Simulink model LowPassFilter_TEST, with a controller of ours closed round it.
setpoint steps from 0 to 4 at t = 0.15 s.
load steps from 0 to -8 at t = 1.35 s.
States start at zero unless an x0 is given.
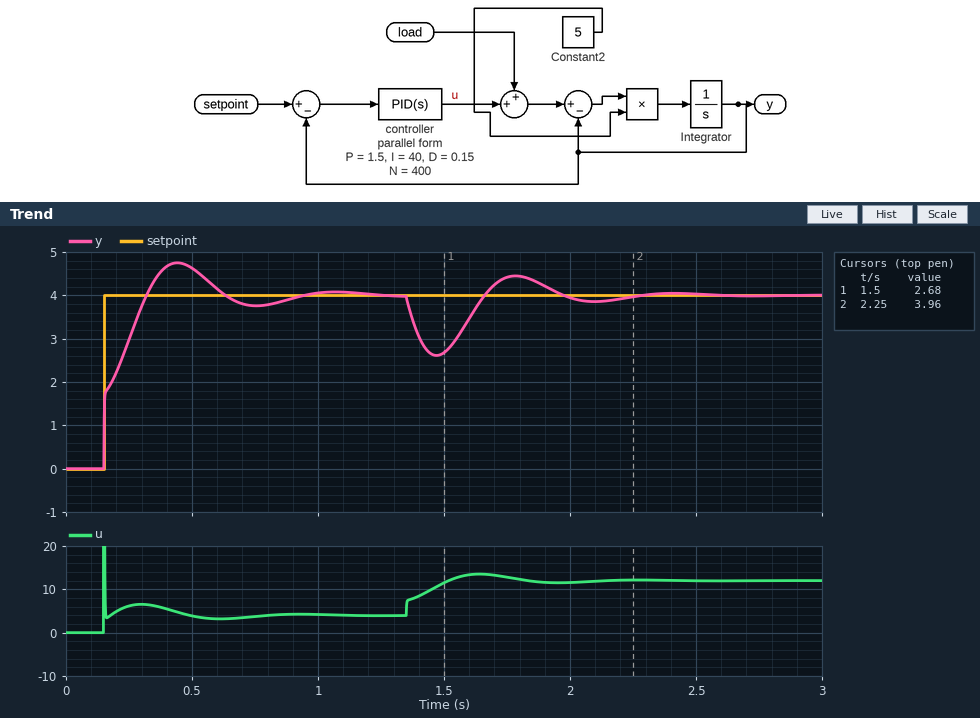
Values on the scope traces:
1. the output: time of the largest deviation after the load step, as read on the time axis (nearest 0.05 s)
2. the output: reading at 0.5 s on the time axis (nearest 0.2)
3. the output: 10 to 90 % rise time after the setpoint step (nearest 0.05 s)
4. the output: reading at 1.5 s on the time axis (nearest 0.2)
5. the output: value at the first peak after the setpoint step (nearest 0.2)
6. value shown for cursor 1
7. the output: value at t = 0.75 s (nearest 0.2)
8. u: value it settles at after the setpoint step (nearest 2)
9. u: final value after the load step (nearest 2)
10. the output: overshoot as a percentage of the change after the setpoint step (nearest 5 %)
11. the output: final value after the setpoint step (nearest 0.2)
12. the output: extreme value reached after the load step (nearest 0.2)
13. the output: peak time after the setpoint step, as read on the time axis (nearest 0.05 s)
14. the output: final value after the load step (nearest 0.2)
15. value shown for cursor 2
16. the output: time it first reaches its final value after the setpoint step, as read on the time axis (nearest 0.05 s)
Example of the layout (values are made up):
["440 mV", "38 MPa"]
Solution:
["1.45 s", "4.6", "0.15 s", "2.6", "4.8", "2.68", "3.8", "4", "12", "20 %", "4.0", "2.6", "0.45 s", "4.0", "3.96", "0.30 s"]
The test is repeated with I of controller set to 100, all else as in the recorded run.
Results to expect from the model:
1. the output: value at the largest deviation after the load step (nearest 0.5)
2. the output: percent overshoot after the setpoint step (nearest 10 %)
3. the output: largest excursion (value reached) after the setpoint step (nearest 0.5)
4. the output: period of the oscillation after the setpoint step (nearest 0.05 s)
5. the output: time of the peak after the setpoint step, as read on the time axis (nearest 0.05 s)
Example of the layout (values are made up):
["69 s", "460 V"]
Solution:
["3.0", "30 %", "5.0", "0.40 s", "0.35 s"]
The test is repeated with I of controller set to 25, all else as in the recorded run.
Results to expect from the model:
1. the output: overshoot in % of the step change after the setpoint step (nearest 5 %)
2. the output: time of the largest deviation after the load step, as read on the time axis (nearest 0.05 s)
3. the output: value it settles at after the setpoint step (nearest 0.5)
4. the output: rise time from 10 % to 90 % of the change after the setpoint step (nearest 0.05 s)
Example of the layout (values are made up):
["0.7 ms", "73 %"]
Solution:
["15 %", "1.50 s", "4.0", "0.20 s"]
